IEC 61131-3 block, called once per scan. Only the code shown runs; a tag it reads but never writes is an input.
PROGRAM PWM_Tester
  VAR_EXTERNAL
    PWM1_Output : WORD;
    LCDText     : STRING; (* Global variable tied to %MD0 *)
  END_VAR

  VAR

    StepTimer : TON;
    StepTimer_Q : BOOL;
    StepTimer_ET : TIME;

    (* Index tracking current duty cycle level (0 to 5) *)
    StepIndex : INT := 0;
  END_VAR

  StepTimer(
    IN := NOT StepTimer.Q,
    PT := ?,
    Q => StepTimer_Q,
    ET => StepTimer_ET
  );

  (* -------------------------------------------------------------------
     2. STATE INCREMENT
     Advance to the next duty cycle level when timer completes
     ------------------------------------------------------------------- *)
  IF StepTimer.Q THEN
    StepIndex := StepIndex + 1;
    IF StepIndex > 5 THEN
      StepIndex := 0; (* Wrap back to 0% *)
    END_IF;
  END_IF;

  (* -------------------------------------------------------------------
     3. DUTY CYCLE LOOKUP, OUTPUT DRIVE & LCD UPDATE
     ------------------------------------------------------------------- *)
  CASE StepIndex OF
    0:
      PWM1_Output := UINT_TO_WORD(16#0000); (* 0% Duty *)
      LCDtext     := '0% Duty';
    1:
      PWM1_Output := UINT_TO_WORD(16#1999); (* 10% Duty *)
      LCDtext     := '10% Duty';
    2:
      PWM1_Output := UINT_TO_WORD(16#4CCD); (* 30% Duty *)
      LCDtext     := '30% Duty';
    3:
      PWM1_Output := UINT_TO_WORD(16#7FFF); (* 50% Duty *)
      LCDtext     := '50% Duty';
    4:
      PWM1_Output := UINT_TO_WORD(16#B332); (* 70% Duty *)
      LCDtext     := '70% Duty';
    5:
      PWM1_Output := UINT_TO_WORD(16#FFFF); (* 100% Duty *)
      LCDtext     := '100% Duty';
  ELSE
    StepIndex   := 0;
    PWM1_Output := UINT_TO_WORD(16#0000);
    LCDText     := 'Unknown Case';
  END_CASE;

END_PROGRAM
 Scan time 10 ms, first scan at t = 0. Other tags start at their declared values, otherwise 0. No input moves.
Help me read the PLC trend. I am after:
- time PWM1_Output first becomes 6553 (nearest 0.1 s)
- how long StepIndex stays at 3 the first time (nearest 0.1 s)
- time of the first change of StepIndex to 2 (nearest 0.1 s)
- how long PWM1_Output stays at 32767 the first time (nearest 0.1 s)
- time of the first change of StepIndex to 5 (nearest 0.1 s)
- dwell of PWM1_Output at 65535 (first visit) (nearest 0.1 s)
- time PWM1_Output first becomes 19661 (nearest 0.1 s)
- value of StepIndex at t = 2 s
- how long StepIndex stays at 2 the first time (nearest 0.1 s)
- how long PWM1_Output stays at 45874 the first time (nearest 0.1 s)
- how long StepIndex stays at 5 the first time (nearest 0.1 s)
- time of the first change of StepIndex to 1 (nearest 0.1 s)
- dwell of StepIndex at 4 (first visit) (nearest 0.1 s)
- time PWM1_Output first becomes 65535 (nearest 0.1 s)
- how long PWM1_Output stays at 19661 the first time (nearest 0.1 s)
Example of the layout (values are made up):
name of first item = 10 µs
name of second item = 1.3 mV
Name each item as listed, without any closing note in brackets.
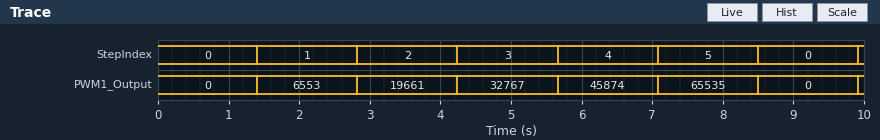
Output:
time PWM1_Output first becomes 6553 = 1.4 s
how long StepIndex stays at 3 the first time = 1.4 s
time of the first change of StepIndex to 2 = 2.8 s
how long PWM1_Output stays at 32767 the first time = 1.4 s
time of the first change of StepIndex to 5 = 7.1 s
dwell of PWM1_Output at 65535 (first visit) = 1.4 s
time PWM1_Output first becomes 19661 = 2.8 s
value of StepIndex at t = 2 s = 1
how long StepIndex stays at 2 the first time = 1.4 s
how long PWM1_Output stays at 45874 the first time = 1.4 s
how long StepIndex stays at 5 the first time = 1.4 s
time of the first change of StepIndex to 1 = 1.4 s
dwell of StepIndex at 4 (first visit) = 1.4 s
time PWM1_Output first becomes 65535 = 7.1 s
how long PWM1_Output stays at 19661 the first time = 1.4 s
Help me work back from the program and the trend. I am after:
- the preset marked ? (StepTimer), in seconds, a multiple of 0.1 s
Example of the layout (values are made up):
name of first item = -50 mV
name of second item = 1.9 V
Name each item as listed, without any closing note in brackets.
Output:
the preset marked ? (StepTimer), in seconds, a multiple of 0.1 s = 1.4 s
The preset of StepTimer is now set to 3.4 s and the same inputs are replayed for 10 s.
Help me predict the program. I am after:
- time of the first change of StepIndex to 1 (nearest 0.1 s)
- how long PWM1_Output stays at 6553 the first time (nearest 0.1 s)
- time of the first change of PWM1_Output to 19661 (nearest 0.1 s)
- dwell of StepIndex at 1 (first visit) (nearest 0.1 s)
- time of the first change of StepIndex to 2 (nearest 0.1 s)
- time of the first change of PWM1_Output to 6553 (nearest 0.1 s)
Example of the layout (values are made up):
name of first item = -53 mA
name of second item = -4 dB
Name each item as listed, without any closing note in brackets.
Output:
time of the first change of StepIndex to 1 = 3.4 s
how long PWM1_Output stays at 6553 the first time = 3.4 s
time of the first change of PWM1_Output to 19661 = 6.8 s
dwell of StepIndex at 1 (first visit) = 3.4 s
time of the first change of StepIndex to 2 = 6.8 s
time of the first change of PWM1_Output to 6553 = 3.4 s
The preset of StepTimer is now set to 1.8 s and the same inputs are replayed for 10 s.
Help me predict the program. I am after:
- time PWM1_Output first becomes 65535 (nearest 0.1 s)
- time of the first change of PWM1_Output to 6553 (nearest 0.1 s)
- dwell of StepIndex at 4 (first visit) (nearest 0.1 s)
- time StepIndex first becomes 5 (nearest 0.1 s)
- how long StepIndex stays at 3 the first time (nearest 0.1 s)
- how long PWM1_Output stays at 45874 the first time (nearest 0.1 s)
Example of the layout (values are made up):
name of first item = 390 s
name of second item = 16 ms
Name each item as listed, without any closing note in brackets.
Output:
time PWM1_Output first becomes 65535 = 9.1 s
time of the first change of PWM1_Output to 6553 = 1.8 s
dwell of StepIndex at 4 (first visit) = 1.8 s
time StepIndex first becomes 5 = 9.1 s
how long StepIndex stays at 3 the first time = 1.8 s
how long PWM1_Output stays at 45874 the first time = 1.8 s
